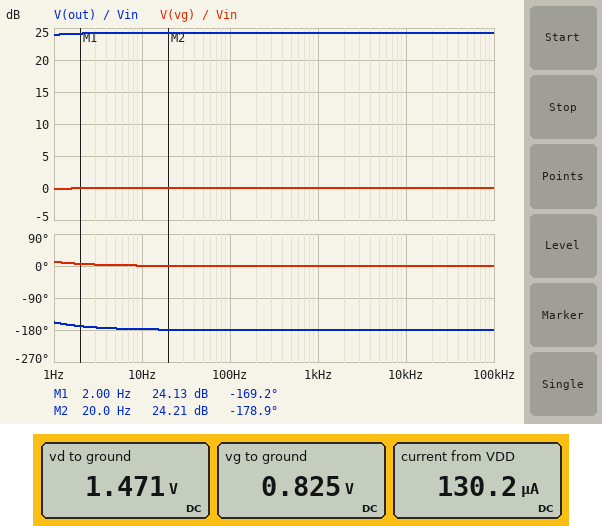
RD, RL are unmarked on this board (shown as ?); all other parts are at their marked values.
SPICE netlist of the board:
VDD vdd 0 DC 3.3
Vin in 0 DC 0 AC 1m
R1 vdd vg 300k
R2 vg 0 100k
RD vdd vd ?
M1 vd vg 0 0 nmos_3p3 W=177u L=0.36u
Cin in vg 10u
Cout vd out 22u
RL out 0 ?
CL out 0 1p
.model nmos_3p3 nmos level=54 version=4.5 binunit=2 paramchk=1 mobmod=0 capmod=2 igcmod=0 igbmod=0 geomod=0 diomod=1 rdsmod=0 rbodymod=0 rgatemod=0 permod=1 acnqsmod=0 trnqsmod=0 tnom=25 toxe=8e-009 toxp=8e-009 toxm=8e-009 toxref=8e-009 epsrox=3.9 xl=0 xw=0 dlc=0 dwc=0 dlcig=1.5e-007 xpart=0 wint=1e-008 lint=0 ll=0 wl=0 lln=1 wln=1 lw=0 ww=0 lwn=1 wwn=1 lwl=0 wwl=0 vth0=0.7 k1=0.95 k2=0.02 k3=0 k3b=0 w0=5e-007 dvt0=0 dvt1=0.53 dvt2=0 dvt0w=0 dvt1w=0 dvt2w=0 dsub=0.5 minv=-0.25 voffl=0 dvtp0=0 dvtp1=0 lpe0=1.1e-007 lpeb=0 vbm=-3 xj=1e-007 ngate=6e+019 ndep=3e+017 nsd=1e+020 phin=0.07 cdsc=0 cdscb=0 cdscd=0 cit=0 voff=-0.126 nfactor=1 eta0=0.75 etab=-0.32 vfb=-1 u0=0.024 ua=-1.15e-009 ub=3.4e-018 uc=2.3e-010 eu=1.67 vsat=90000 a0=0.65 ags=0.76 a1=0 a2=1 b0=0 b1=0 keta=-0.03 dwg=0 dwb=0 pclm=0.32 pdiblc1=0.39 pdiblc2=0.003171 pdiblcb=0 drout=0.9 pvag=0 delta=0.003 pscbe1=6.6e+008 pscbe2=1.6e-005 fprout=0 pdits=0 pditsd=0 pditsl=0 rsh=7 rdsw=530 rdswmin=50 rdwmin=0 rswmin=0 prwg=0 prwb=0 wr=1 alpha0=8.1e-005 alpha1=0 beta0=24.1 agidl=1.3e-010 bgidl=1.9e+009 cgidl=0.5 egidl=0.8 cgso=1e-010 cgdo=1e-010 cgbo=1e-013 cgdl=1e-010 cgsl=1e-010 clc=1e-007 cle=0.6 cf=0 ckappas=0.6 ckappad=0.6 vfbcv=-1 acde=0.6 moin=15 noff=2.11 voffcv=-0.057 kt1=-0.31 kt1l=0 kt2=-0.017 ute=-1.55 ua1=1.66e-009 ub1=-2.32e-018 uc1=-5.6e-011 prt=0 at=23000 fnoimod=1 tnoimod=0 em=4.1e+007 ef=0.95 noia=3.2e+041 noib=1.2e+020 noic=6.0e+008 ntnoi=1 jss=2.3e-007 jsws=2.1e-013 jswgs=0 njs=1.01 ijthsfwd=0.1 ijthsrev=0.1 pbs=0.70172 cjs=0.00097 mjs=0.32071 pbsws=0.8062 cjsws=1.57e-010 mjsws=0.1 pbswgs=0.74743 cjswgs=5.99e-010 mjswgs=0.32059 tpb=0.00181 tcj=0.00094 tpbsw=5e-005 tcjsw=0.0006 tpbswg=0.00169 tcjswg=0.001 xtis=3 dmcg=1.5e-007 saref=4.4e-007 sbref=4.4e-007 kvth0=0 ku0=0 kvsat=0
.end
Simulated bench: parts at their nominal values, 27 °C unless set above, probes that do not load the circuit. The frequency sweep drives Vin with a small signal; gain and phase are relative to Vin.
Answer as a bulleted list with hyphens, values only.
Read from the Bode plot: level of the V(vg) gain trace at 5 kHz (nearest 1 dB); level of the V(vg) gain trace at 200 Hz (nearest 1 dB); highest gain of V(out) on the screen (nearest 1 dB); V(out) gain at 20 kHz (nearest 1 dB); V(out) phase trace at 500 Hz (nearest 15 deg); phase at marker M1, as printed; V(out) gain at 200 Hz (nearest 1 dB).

- 0 dB
- 0 dB
- 24 dB
- 24 dB
- -180 deg
- -169.2 deg
- 24 dB
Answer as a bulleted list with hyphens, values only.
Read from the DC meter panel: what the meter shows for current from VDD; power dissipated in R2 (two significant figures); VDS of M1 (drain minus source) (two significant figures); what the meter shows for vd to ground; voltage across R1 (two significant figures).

- 130.2 µA
- 6.8 µW
- 1.5 V
- 1.471 V
- 2.5 V
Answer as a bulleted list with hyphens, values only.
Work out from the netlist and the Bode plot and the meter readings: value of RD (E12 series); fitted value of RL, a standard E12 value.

- 15 kΩ
- 33 kΩ
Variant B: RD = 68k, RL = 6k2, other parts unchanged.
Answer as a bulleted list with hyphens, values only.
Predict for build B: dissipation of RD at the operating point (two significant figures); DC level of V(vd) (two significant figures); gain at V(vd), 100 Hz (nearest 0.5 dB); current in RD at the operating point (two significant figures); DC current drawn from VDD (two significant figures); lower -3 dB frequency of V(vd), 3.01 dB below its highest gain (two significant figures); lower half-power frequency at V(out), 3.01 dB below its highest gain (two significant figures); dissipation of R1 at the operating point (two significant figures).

- 160 µW
- 28 mV
- -7.0 dB
- 48 µA
- 56 µA
- 190 mHz
- 1.1 Hz
- 20 µW
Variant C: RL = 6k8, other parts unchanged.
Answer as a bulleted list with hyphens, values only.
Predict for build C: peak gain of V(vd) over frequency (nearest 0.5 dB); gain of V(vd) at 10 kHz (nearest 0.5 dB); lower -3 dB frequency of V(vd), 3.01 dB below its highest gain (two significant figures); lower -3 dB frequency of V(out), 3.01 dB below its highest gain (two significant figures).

- 23.5 dB
- 18.5 dB
- 120 mHz
- 490 mHz
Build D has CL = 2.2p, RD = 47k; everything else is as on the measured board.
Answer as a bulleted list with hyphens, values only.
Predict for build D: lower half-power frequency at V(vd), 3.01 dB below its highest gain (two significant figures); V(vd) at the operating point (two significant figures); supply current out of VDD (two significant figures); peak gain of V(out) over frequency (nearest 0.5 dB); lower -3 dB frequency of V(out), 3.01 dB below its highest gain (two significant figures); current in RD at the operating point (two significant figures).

- 200 mHz
- 48 mV
- 77 µA
- 2.0 dB
- 330 mHz
- 69 µA
